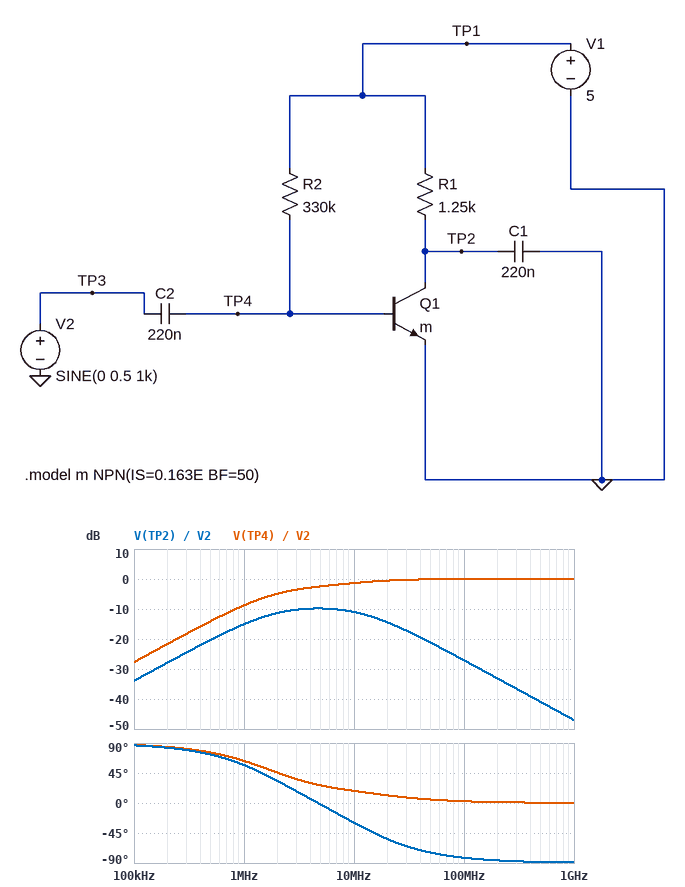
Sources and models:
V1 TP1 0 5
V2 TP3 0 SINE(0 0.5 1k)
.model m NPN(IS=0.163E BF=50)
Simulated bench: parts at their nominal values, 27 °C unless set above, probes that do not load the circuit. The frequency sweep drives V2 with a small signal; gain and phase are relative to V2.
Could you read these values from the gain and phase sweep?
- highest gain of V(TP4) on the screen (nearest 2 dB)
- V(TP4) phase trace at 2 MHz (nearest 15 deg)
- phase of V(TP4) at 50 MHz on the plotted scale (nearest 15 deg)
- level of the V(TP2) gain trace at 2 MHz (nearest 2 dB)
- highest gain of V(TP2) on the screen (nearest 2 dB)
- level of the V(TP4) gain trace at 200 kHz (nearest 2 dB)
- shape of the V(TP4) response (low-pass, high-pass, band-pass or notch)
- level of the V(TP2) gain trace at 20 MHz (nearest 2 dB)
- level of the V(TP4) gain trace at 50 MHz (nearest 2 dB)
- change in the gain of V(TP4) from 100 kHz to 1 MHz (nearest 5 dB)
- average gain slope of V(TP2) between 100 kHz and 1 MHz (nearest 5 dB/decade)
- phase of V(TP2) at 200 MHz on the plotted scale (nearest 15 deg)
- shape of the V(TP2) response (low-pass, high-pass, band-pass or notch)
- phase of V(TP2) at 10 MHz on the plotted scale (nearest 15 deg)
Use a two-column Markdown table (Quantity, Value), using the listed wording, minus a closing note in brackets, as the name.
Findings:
| Quantity | Value |
|---|---|
| highest gain of V(TP4) on the screen | 0 dB |
| V(TP4) phase trace at 2 MHz | 45 deg |
| phase of V(TP4) at 50 MHz on the plotted scale | 0 deg |
| level of the V(TP2) gain trace at 2 MHz | -12 dB |
| highest gain of V(TP2) on the screen | -10 dB |
| level of the V(TP4) gain trace at 200 kHz | -22 dB |
| shape of the V(TP4) response | high-pass |
| level of the V(TP2) gain trace at 20 MHz | -14 dB |
| level of the V(TP4) gain trace at 50 MHz | 0 dB |
| change in the gain of V(TP4) from 100 kHz to 1 MHz | 20 dB |
| average gain slope of V(TP2) between 100 kHz and 1 MHz | 20 dB/decade |
| phase of V(TP2) at 200 MHz on the plotted scale | -90 deg |
| shape of the V(TP2) response | band-pass |
| phase of V(TP2) at 10 MHz on the plotted scale | -30 deg |
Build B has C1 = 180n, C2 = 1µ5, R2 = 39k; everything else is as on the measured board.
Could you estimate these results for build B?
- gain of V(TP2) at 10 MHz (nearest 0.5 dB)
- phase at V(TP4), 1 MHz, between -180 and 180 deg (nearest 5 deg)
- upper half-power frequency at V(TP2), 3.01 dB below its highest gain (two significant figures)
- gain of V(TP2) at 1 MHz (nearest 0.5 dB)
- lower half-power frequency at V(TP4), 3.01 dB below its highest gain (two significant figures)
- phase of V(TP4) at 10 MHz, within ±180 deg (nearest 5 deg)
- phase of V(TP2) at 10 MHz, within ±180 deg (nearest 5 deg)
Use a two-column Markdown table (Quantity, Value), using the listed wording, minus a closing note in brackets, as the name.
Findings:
| Quantity | Value |
|---|---|
| gain of V(TP2) at 10 MHz | -9.0 dB |
| phase at V(TP4), 1 MHz, between -180 and 180 deg | 20 deg |
| upper half-power frequency at V(TP2), 3.01 dB below its highest gain | 12 MHz |
| gain of V(TP2) at 1 MHz | -7.0 dB |
| lower half-power frequency at V(TP4), 3.01 dB below its highest gain | 370 kHz |
| phase of V(TP4) at 10 MHz, within ±180 deg | 5 deg |
| phase of V(TP2) at 10 MHz, within ±180 deg | -40 deg |
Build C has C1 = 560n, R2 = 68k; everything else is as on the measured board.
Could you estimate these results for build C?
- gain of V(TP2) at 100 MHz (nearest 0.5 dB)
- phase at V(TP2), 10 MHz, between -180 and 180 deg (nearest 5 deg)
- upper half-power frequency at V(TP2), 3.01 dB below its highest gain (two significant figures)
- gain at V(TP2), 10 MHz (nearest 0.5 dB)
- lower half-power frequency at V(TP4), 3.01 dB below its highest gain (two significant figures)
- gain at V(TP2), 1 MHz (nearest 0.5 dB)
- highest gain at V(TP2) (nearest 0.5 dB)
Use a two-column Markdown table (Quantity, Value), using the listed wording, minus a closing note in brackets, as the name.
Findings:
| Quantity | Value |
|---|---|
| gain of V(TP2) at 100 MHz | -35.0 dB |
| phase at V(TP2), 10 MHz, between -180 and 180 deg | -50 deg |
| upper half-power frequency at V(TP2), 3.01 dB below its highest gain | 9.2 MHz |
| gain at V(TP2), 10 MHz | -17.0 dB |
| lower half-power frequency at V(TP4), 3.01 dB below its highest gain | 5.2 MHz |
| gain at V(TP2), 1 MHz | -16.0 dB |
| highest gain at V(TP2) | -13.5 dB |
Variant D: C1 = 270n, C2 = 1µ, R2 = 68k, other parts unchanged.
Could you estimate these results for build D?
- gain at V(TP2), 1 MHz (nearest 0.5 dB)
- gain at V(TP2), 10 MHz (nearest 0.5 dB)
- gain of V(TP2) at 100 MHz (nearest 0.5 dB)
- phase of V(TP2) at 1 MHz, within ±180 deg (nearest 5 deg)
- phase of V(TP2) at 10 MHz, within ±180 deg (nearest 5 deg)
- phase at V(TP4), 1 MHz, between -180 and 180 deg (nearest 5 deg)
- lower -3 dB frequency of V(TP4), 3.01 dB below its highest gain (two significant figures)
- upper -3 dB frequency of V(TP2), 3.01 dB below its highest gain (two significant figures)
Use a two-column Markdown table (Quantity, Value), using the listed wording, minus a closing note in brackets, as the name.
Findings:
| Quantity | Value |
|---|---|
| gain at V(TP2), 1 MHz | -8.0 dB |
| gain at V(TP2), 10 MHz | -11.0 dB |
| gain of V(TP2) at 100 MHz | -29.0 dB |
| phase of V(TP2) at 1 MHz, within ±180 deg | 20 deg |
| phase of V(TP2) at 10 MHz, within ±180 deg | -50 deg |
| phase at V(TP4), 1 MHz, between -180 and 180 deg | 25 deg |
| lower -3 dB frequency of V(TP4), 3.01 dB below its highest gain | 580 kHz |
| upper -3 dB frequency of V(TP2), 3.01 dB below its highest gain | 8.9 MHz |
